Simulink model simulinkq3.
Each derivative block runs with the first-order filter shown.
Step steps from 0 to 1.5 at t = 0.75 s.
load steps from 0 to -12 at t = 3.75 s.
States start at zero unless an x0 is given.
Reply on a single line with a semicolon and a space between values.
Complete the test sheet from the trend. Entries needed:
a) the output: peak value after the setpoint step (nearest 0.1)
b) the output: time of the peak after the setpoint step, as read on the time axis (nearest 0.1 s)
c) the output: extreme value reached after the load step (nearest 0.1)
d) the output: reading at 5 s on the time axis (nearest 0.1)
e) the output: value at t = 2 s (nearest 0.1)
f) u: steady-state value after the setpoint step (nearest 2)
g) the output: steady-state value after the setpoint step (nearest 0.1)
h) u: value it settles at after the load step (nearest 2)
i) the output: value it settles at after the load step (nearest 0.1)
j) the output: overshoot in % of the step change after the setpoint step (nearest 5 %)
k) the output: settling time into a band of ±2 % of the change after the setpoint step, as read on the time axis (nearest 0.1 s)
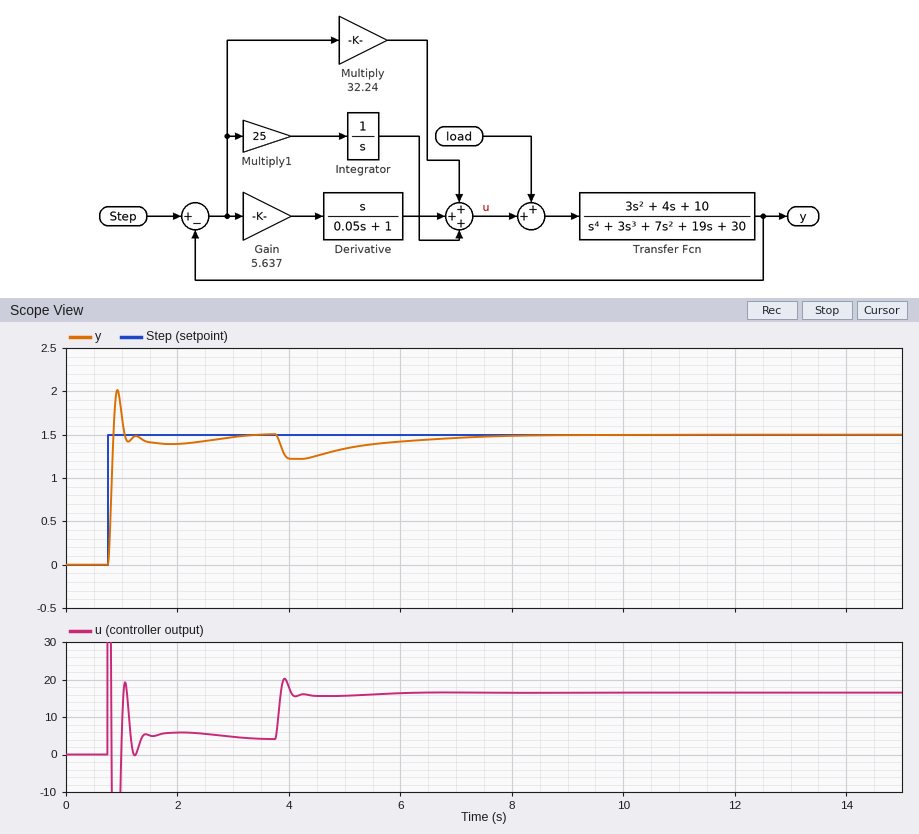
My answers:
2.0; 0.9 s; 1.2; 1.3; 1.4; 4; 1.5; 16; 1.5; 35 %; 3.0 s
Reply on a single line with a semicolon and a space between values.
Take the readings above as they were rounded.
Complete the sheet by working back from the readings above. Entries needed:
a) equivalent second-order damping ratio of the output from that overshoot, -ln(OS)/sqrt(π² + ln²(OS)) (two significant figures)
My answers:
0.32
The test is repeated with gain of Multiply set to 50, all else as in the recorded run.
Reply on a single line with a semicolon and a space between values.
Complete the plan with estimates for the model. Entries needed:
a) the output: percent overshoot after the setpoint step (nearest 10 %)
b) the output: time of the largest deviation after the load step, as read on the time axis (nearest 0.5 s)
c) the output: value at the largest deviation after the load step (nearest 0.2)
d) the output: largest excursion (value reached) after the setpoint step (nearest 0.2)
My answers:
40 %; 4.0 s; 1.2; 2.2
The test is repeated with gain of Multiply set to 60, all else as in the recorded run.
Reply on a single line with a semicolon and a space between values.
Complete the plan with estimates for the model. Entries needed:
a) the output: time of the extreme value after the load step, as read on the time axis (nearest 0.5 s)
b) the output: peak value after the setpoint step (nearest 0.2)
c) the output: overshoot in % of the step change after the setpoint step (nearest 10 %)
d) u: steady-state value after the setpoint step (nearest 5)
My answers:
4.0 s; 2.2; 50 %; 5
